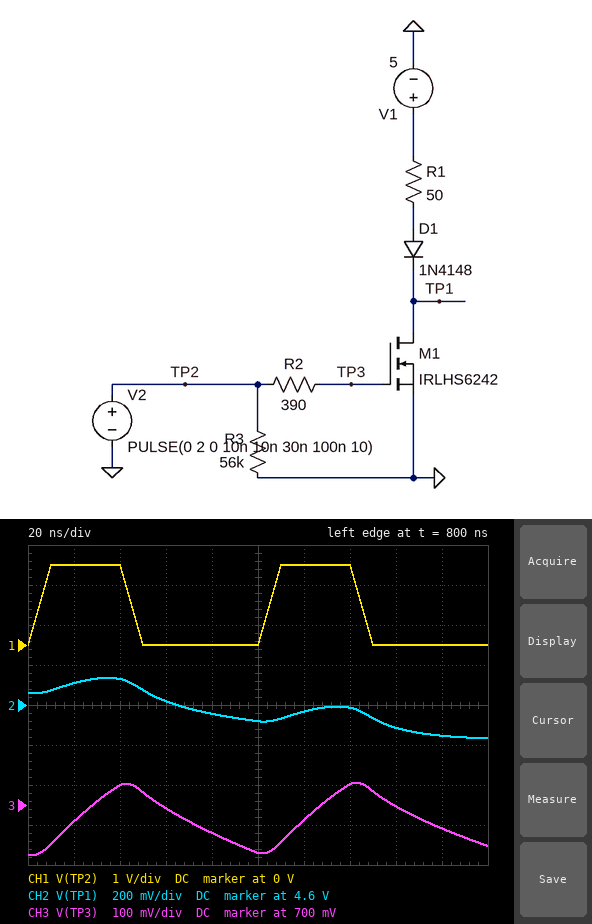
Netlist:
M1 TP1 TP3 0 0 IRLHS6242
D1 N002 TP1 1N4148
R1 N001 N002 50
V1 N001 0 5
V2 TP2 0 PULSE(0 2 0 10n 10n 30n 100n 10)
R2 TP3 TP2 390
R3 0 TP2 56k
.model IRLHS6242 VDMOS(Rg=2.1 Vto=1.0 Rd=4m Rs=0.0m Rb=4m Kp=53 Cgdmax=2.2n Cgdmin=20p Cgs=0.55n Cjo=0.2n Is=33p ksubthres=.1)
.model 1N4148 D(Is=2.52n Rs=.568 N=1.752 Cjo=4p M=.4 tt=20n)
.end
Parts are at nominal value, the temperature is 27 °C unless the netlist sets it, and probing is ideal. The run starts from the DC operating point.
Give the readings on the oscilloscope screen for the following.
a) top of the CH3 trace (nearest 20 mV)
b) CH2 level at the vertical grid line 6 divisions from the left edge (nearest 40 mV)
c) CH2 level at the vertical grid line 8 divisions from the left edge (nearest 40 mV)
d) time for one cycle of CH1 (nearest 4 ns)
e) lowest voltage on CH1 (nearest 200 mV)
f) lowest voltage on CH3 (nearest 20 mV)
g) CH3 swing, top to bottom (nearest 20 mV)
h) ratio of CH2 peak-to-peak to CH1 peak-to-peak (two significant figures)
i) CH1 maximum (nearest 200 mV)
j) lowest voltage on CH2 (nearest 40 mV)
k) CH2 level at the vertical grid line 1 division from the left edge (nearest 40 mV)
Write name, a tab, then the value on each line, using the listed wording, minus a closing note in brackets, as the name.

top of the CH3 trace	760 mV
CH2 level at the vertical grid line 6 divisions from the left edge	4.56 V
CH2 level at the vertical grid line 8 divisions from the left edge	4.48 V
time for one cycle of CH1	100 ns
lowest voltage on CH1	0 V
lowest voltage on CH3	580 mV
CH3 swing, top to bottom	180 mV
ratio of CH2 peak-to-peak to CH1 peak-to-peak	0.15
CH1 maximum	2.0 V
lowest voltage on CH2	4.44 V
CH2 level at the vertical grid line 1 division from the left edge	4.72 V
